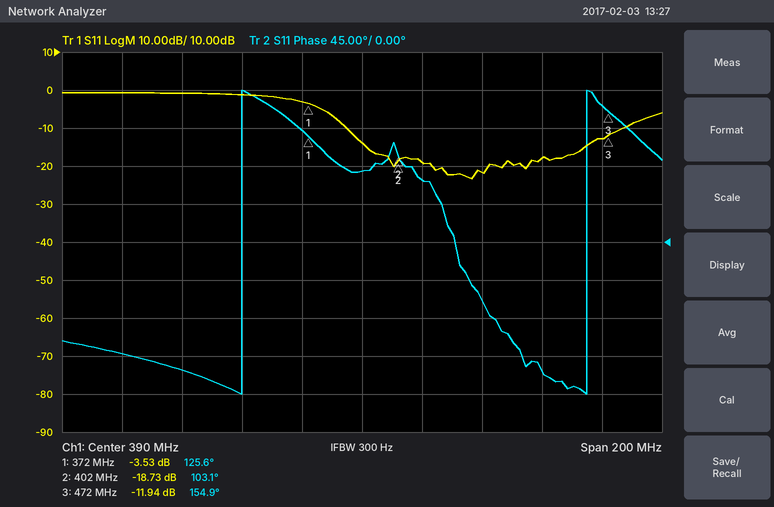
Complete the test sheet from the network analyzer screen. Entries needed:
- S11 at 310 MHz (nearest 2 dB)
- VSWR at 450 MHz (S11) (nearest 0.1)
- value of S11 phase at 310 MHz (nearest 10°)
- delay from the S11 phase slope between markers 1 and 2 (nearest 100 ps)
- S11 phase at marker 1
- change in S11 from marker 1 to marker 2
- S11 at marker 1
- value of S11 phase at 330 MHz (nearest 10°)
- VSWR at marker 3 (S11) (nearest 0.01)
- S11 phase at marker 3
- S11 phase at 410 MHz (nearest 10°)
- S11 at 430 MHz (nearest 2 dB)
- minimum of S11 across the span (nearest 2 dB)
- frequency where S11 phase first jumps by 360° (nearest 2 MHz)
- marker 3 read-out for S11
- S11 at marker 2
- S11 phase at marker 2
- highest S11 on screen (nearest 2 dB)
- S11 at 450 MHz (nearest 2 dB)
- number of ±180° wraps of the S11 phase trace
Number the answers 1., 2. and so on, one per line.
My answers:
1. 0 dB
2. 1.3
3. -130°
4. 2.1 ns
5. 125.6°
6. -15.20 dB
7. -3.53 dB
8. -150°
9. 1.68
10. 154.9°
11. 70°
12. -22 dB
13. -24 dB
14. 350 MHz
15. -11.94 dB
16. -18.73 dB
17. 103.1°
18. 0 dB
19. -18 dB
20. 2
